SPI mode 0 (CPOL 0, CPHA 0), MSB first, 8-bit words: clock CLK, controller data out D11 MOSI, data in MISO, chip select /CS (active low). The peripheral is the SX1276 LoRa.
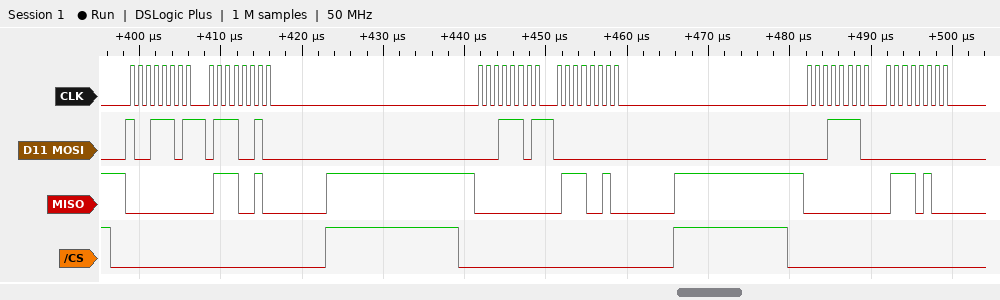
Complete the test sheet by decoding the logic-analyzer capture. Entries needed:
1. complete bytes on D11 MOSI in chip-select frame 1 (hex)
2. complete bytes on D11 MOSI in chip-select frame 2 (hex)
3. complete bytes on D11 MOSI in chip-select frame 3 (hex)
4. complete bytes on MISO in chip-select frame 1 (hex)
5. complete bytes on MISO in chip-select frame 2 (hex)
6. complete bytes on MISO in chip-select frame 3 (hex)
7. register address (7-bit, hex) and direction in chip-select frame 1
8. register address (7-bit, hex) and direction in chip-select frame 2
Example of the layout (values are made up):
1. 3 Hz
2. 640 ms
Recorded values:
1. 0x9D 0x72
2. 0x1D 0x00
3. 0x1E 0x00
4. 0x00 0x72
5. 0x00 0x72
6. 0x00 0x74
7. 0x1D write
8. 0x1D read
